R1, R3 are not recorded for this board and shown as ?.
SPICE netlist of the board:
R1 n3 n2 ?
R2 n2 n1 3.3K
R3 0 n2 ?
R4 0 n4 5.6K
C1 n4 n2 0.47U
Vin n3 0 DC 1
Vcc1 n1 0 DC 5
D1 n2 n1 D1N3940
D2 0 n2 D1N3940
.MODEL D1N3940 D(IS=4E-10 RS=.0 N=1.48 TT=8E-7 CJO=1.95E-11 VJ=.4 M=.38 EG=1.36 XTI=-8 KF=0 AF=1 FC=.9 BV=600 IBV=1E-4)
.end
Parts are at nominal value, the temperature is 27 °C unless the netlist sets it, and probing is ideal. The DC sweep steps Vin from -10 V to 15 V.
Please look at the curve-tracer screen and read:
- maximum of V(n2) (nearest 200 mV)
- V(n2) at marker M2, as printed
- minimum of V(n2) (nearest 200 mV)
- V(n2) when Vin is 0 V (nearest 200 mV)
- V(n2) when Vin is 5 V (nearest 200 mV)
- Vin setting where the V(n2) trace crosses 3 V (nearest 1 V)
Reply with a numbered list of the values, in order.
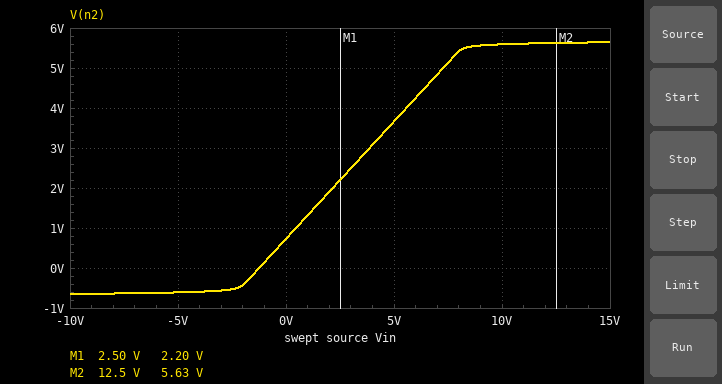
1. 5.6 V
2. 5.63 V
3. -600 mV
4. 800 mV
5. 3.6 V
6. 4 V
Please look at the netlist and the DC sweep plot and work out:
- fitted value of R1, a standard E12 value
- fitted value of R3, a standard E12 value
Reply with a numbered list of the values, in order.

1. 820 Ω
2. 1.8 kΩ
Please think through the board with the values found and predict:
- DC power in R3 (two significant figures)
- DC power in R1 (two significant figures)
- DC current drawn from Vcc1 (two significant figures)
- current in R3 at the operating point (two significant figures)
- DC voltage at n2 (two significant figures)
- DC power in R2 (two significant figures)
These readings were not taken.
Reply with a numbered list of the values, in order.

1. 960 µW
2. 120 µW
3. 1.1 mA
4. 730 µA
5. 1.3 V
6. 4.1 mW
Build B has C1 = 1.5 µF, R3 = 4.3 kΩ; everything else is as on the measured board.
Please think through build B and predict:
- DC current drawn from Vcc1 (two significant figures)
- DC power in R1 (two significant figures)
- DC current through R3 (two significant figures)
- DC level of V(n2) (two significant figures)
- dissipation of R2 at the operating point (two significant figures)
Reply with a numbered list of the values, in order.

1. 1.0 mA
2. 380 µW
3. 360 µA
4. 1.6 V
5. 3.6 mW
